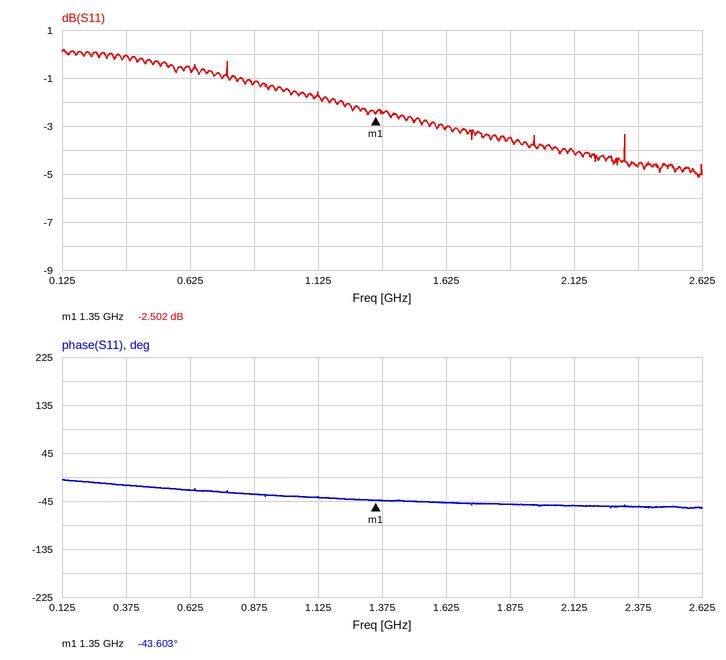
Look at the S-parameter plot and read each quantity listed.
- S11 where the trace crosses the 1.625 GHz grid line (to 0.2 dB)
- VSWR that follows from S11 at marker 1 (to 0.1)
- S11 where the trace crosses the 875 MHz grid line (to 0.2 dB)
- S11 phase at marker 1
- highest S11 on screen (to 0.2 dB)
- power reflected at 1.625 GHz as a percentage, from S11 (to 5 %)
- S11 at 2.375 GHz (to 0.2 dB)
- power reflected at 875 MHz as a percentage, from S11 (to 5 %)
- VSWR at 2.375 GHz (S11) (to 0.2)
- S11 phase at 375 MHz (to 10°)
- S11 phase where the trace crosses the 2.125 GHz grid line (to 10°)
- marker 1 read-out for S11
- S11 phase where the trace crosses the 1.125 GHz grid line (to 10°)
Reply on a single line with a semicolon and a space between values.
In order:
-3.0 dB; 7.0; -1.2 dB; -43.603°; 0.2 dB; 50 %; -4.6 dB; 75 %; 3.8; -20°; -50°; -2.502 dB; -40°
